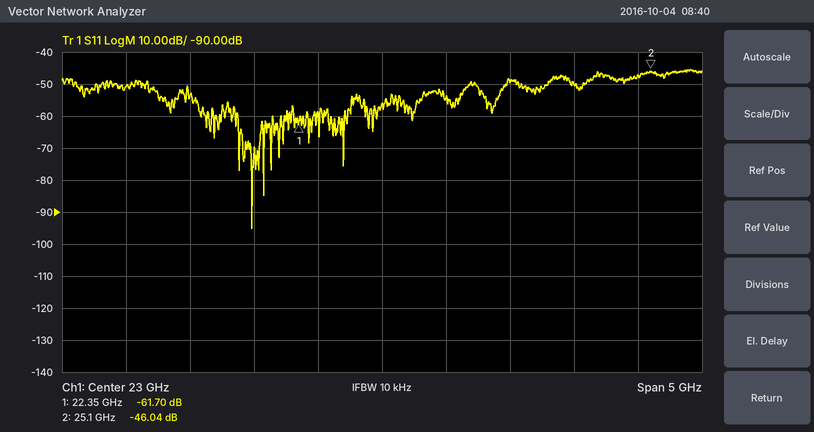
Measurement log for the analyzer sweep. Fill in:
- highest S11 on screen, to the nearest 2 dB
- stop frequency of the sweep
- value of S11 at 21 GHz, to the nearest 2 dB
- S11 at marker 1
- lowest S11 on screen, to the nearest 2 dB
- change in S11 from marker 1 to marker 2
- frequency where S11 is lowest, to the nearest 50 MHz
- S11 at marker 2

-46 dB
25.5 GHz
-50 dB
-61.70 dB
-96 dB
15.66 dB
22.00 GHz
-46.04 dB
